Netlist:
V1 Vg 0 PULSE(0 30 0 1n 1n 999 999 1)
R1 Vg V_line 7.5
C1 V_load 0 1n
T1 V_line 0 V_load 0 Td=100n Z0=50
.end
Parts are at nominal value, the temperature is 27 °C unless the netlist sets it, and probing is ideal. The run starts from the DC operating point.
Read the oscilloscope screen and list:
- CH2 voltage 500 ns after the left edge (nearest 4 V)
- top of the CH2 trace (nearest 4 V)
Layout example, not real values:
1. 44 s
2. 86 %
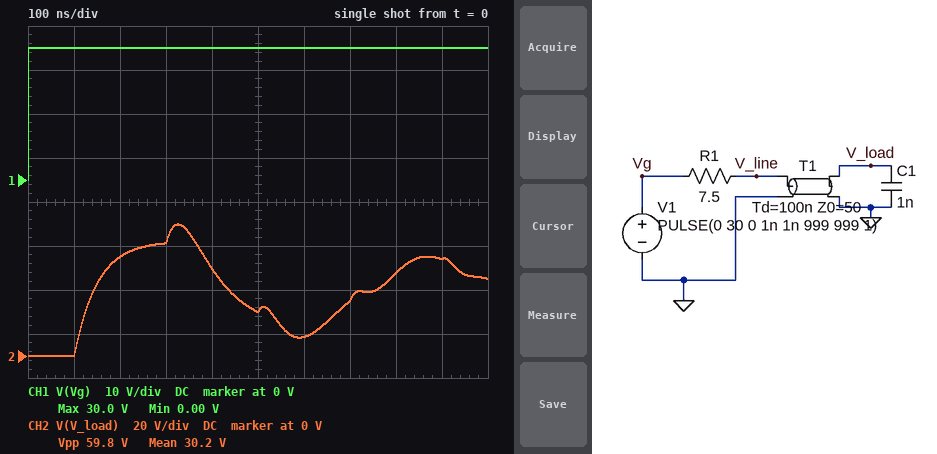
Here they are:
1. 20 V
2. 60 V
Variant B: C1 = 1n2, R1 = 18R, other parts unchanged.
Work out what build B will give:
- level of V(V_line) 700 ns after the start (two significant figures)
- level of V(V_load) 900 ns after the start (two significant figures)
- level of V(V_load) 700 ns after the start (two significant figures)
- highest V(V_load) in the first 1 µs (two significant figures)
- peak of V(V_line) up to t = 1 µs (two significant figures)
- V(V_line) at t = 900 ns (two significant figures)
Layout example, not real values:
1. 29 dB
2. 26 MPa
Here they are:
1. 28 V
2. 33 V
3. 25 V
4. 48 V
5. 36 V
6. 29 V
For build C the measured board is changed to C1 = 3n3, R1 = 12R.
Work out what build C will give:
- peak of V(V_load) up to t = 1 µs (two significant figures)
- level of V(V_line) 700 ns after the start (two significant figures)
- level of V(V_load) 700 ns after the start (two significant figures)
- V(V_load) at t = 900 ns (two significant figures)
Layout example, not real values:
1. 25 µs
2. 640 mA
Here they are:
1. 47 V
2. 35 V
3. 30 V
4. 21 V
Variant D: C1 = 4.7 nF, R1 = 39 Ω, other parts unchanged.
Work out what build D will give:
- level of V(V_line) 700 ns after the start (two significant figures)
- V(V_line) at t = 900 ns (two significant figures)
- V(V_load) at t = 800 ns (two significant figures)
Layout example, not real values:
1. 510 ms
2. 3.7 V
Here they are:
1. 29 V
2. 30 V
3. 30 V
